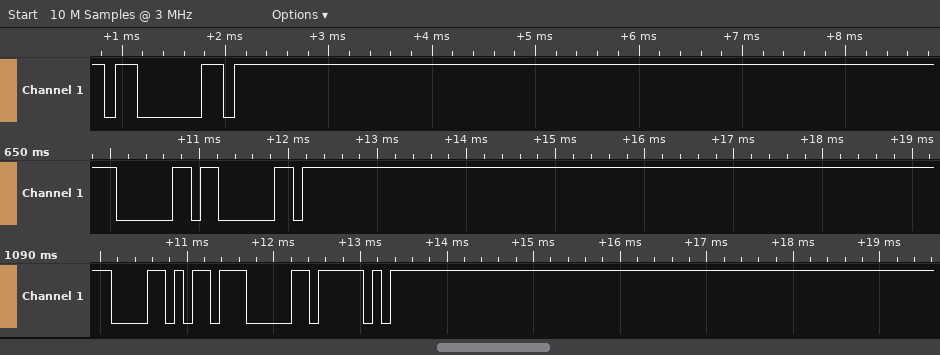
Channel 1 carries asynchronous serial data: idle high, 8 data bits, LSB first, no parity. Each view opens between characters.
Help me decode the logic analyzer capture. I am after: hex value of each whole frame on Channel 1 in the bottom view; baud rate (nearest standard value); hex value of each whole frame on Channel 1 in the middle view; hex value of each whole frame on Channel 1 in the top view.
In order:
58, 07, 5F
9600 baud
60, 60
03, FF
